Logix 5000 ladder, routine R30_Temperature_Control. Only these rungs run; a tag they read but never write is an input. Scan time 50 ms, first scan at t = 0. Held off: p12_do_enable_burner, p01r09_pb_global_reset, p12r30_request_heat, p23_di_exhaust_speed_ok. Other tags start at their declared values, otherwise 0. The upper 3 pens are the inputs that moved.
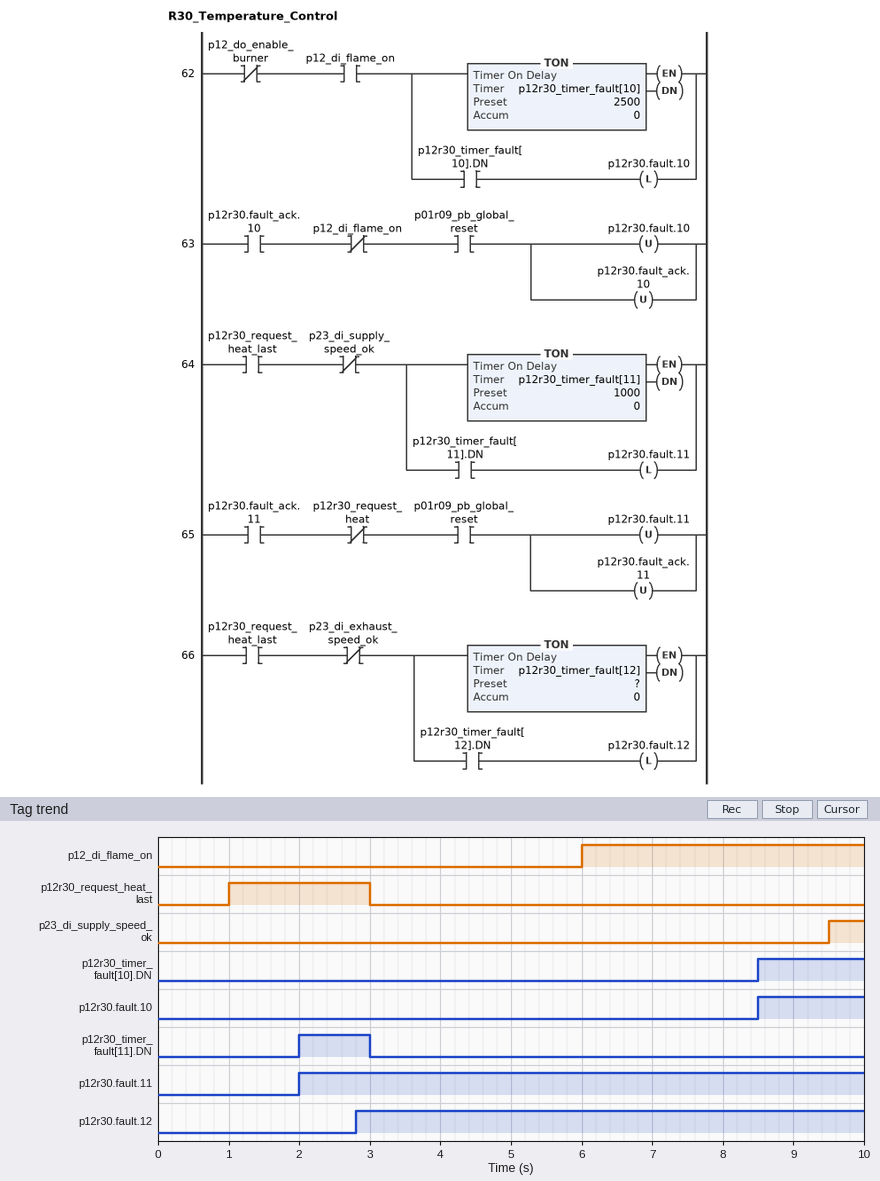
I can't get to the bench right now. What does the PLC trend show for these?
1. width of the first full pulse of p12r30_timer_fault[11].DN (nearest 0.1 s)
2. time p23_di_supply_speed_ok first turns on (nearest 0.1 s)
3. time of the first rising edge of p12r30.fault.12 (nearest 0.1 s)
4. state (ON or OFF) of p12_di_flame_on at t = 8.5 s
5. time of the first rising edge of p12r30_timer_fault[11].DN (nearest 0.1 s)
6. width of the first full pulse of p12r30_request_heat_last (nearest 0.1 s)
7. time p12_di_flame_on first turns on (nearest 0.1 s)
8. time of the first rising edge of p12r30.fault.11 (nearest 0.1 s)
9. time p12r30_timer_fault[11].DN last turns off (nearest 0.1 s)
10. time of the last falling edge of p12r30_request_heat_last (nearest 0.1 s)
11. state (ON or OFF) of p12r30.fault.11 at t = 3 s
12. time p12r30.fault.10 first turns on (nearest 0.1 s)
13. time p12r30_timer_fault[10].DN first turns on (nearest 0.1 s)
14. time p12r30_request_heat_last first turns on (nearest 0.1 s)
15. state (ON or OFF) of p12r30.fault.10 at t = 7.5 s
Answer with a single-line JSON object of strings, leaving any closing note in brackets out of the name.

{"width of the first full pulse of p12r30_timer_fault[11].DN": "1.0 s", "time p23_di_supply_speed_ok first turns on": "9.5 s", "time of the first rising edge of p12r30.fault.12": "2.8 s", "state (ON or OFF) of p12_di_flame_on at t = 8.5 s": "ON", "time of the first rising edge of p12r30_timer_fault[11].DN": "2.0 s", "width of the first full pulse of p12r30_request_heat_last": "2.0 s", "time p12_di_flame_on first turns on": "6.0 s", "time of the first rising edge of p12r30.fault.11": "2.0 s", "time p12r30_timer_fault[11].DN last turns off": "3.0 s", "time of the last falling edge of p12r30_request_heat_last": "3.0 s", "state (ON or OFF) of p12r30.fault.11 at t = 3 s": "ON", "time p12r30.fault.10 first turns on": "8.5 s", "time p12r30_timer_fault[10].DN first turns on": "8.5 s", "time p12r30_request_heat_last first turns on": "1.0 s", "state (ON or OFF) of p12r30.fault.10 at t = 7.5 s": "OFF"}
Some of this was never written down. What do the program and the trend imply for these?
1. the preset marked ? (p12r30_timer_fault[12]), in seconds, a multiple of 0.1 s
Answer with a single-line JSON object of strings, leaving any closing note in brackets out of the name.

{"the preset marked ? (p12r30_timer_fault[12]), in seconds, a multiple of 0.1 s": "1.8 s"}
